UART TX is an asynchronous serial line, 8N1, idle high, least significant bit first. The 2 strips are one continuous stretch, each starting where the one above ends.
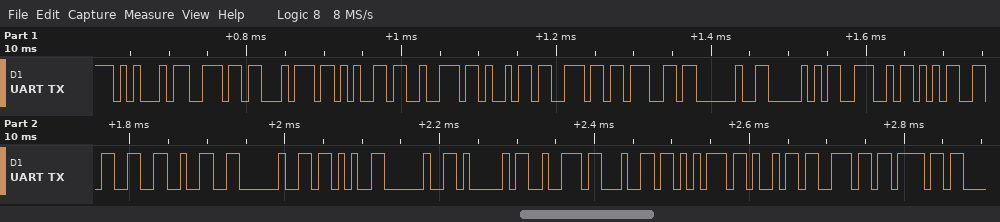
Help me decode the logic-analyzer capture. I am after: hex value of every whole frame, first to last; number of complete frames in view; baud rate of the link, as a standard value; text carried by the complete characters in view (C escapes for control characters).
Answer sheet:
45 6E 74 65 72 69 6E 67 20 50 4E 35 33 32 20 2B 20 41 72 64 75 69 6E 6F
24
115200 baud
"Entering PN532 + Arduino"
